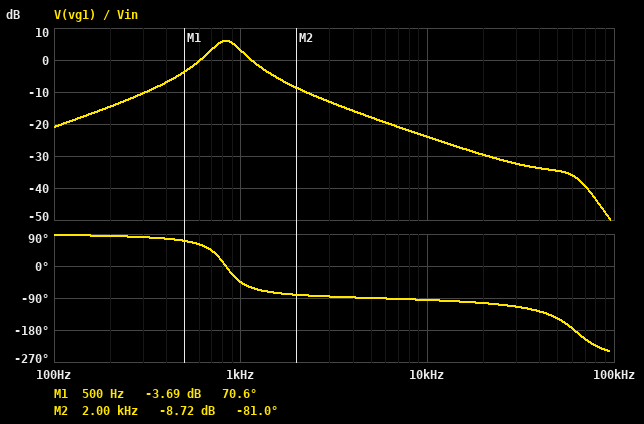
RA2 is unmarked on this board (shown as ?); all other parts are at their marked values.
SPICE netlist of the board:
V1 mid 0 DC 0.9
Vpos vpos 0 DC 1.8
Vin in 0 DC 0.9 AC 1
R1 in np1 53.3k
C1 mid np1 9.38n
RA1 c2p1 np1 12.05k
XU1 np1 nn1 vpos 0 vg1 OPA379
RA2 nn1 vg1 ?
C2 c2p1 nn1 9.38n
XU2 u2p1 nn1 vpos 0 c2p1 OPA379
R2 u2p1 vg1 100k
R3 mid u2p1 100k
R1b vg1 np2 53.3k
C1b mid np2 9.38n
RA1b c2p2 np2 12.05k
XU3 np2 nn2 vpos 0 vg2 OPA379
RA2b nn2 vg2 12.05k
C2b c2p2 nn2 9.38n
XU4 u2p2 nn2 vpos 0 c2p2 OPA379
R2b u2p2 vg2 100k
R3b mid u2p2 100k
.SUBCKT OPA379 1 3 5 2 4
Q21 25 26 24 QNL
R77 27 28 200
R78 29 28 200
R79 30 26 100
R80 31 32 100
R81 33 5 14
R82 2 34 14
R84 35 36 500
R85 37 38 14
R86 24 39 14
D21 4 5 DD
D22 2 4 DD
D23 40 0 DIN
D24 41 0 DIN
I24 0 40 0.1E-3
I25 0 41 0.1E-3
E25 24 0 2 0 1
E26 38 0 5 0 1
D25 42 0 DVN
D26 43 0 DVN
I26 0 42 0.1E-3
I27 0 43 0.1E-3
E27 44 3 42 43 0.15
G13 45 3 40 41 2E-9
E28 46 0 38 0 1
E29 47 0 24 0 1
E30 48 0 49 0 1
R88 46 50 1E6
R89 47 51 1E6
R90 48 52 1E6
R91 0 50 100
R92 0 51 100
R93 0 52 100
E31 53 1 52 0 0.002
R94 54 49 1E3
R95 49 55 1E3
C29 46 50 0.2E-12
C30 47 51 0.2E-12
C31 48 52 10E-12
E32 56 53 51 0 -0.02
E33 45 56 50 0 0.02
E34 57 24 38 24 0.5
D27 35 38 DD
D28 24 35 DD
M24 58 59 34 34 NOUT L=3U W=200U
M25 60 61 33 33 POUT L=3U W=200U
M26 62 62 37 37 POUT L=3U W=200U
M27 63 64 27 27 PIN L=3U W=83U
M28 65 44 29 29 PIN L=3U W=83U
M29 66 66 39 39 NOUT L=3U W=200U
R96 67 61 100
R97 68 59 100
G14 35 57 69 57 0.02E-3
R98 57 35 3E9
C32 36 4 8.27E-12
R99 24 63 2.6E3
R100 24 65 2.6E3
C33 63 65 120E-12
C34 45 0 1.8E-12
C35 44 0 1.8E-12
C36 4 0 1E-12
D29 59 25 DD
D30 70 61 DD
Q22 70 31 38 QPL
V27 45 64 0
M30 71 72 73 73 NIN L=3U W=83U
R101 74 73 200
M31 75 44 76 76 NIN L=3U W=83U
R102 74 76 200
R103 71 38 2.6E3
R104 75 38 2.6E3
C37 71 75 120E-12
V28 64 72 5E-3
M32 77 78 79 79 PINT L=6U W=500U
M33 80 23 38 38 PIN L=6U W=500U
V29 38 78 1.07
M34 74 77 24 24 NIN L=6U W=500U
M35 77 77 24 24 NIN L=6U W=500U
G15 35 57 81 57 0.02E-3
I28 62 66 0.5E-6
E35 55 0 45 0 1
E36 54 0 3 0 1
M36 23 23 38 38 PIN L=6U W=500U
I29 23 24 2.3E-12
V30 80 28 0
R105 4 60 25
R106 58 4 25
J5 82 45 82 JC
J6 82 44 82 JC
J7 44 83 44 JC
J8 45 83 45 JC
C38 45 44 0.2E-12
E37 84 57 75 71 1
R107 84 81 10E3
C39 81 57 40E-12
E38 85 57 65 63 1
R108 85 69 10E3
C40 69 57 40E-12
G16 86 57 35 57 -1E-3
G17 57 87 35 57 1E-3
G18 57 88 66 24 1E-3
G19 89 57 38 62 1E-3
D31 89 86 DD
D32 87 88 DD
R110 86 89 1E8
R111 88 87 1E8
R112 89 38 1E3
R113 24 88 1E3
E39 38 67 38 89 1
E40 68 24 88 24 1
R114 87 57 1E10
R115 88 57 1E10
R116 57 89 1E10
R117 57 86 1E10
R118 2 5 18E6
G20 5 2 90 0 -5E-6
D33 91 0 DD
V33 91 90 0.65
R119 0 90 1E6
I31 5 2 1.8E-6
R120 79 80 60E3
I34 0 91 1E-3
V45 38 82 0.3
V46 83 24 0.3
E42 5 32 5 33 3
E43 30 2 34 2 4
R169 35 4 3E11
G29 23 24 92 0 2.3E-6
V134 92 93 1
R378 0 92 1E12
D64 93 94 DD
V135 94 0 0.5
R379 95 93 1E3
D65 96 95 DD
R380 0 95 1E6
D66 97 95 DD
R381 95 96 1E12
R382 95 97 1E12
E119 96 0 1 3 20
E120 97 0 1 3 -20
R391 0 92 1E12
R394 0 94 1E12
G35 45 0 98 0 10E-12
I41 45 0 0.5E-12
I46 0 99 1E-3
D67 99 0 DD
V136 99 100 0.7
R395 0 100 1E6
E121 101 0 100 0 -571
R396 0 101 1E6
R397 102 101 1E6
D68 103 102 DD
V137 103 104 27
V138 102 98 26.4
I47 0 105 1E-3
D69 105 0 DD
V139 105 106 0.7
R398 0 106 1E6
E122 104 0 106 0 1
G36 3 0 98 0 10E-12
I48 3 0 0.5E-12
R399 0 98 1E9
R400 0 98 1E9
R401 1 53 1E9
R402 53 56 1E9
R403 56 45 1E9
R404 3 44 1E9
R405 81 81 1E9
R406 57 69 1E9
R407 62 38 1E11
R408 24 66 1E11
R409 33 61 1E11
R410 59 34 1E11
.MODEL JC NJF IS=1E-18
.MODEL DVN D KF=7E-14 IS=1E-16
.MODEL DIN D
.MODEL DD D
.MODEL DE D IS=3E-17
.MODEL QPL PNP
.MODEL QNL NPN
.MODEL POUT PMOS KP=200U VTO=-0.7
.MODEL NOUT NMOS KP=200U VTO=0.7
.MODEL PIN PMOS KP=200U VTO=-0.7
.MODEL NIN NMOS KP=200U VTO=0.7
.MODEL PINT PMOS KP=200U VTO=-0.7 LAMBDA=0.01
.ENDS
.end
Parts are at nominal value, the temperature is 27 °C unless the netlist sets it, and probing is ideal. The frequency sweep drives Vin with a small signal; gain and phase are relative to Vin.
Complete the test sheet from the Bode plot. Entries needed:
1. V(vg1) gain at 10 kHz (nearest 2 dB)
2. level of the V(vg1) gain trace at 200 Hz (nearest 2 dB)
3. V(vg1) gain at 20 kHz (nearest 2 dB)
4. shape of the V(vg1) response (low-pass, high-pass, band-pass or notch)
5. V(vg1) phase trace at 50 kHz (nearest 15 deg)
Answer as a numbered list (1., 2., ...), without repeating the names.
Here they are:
1. -24 dB
2. -14 dB
3. -30 dB
4. band-pass
5. -150 deg
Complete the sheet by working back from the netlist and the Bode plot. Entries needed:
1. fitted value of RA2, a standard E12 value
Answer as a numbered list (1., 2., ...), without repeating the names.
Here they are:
1. 33 kΩ
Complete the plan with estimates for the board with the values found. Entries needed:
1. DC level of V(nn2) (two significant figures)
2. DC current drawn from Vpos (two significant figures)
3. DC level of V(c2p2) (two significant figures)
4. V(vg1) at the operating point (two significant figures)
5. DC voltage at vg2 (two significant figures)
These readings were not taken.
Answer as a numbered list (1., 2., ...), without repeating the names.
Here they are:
1. 890 mV
2. 9.4 µA
3. 900 mV
4. 890 mV
5. 890 mV
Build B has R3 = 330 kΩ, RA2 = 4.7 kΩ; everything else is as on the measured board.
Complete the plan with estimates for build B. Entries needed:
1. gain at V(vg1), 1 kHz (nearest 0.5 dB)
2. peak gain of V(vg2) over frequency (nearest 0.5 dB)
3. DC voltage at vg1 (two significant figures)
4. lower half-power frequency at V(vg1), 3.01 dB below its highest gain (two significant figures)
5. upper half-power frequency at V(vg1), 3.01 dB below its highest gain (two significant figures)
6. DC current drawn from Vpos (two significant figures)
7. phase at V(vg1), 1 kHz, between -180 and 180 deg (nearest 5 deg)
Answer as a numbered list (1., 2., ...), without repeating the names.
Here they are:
1. -6.5 dB
2. 6.0 dB
3. 880 mV
4. 1.1 kHz
5. 1.6 kHz
6. 9.3 µA
7. 60 deg
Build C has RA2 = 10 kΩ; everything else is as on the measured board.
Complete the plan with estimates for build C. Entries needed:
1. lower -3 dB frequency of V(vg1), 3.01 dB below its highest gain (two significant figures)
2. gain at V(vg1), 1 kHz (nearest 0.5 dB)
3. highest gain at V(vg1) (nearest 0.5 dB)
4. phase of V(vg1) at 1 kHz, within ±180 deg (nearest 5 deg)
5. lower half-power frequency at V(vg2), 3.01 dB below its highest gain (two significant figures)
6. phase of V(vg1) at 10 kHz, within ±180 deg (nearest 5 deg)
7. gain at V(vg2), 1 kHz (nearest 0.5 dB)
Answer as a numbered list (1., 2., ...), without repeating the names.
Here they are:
1. 1.4 kHz
2. -6.5 dB
3. 6.5 dB
4. 75 deg
5. 1.3 kHz
6. -100 deg
7. -10.0 dB
